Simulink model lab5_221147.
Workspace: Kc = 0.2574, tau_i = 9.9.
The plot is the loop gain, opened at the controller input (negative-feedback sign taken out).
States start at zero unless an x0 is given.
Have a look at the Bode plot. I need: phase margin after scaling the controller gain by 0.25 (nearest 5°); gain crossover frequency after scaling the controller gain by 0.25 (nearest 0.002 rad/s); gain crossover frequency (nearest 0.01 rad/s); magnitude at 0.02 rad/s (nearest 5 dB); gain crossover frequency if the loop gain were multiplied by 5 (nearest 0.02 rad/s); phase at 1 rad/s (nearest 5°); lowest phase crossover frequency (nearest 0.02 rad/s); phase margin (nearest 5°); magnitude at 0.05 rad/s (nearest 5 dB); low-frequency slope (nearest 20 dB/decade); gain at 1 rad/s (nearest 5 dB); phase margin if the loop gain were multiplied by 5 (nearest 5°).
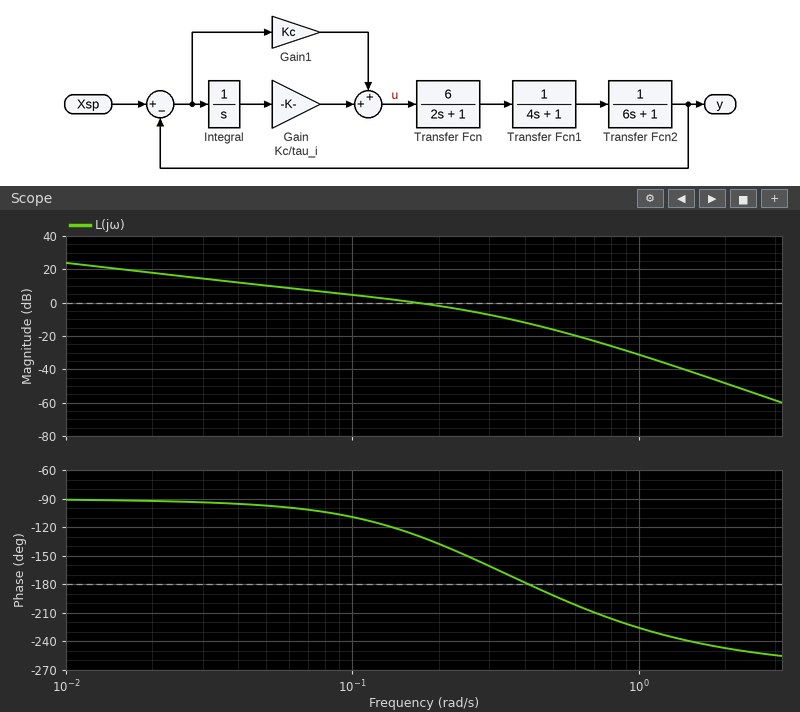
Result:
85°
0.040 rad/s
0.17 rad/s
20 dB
0.44 rad/s
-225°
0.42 rad/s
50°
10 dB
-20 dB/decade
-30 dB
-5°
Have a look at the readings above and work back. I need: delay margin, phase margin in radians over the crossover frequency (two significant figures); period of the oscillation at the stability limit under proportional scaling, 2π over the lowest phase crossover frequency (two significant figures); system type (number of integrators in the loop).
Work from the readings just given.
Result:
5.1 s
15 s
1
